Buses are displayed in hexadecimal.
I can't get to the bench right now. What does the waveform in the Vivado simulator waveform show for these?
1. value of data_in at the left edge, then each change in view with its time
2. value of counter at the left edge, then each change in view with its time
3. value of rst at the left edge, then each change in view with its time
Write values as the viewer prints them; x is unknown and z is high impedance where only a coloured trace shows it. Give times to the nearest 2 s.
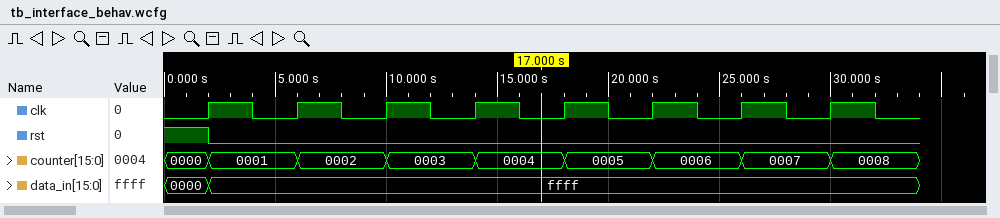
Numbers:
0000, ffff at 2 s
0000, 0001 at 2 s, 0002 at 6 s, 0003 at 10 s, 0004 at 14 s, 0005 at 18 s, 0006 at 22 s, 0007 at 26 s, 0008 at 30 s
1, 0 at 2 s
